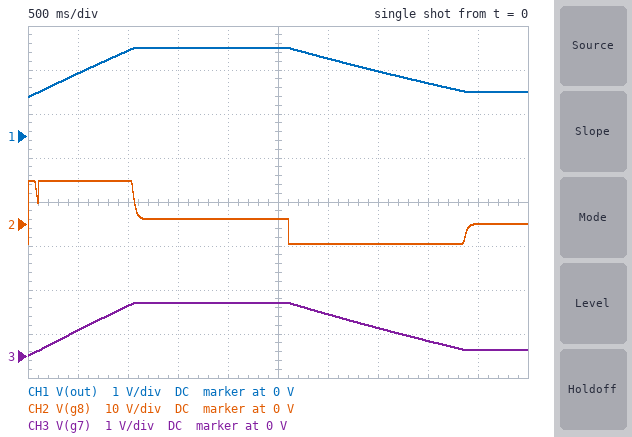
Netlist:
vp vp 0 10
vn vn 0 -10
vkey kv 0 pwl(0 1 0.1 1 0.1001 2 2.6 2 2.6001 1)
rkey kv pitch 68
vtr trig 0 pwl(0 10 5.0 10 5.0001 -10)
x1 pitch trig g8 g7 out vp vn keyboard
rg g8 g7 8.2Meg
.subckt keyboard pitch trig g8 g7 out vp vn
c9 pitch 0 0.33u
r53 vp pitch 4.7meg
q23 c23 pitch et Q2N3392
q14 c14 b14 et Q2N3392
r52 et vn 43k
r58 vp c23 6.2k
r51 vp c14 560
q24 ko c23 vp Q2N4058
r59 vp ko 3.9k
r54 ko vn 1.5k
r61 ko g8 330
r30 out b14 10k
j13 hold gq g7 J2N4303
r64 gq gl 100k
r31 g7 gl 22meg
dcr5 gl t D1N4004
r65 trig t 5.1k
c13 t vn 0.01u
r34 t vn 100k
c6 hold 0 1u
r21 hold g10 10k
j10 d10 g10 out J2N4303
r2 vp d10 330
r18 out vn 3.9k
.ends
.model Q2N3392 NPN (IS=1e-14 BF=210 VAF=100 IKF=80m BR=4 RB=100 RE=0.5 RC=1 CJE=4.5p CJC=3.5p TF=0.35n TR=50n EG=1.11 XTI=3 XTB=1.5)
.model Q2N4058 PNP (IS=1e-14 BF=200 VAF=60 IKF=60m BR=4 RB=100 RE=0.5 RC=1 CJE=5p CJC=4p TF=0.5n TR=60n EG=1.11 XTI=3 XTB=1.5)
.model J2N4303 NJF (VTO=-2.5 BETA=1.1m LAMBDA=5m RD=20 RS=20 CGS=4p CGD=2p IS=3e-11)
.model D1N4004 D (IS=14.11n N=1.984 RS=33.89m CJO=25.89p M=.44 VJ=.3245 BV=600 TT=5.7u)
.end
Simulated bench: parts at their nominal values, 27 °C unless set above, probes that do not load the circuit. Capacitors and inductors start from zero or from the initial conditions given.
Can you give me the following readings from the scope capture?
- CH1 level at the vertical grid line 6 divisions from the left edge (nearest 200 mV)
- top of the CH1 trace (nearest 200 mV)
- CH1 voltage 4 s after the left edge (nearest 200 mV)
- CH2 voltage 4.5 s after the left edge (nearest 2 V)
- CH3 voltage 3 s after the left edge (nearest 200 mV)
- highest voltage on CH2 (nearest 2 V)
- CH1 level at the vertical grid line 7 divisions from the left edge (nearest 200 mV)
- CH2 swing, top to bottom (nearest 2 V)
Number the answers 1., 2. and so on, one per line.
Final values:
1. 1.8 V
2. 2.0 V
3. 1.2 V
4. 0 V
5. 1.0 V
6. 10 V
7. 1.4 V
8. 14 V
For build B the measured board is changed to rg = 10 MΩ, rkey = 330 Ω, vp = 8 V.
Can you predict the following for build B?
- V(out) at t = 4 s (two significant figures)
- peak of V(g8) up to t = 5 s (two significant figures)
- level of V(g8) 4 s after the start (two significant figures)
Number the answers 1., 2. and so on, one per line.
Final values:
1. 1.3 V
2. 7.9 V
3. -5.0 V
